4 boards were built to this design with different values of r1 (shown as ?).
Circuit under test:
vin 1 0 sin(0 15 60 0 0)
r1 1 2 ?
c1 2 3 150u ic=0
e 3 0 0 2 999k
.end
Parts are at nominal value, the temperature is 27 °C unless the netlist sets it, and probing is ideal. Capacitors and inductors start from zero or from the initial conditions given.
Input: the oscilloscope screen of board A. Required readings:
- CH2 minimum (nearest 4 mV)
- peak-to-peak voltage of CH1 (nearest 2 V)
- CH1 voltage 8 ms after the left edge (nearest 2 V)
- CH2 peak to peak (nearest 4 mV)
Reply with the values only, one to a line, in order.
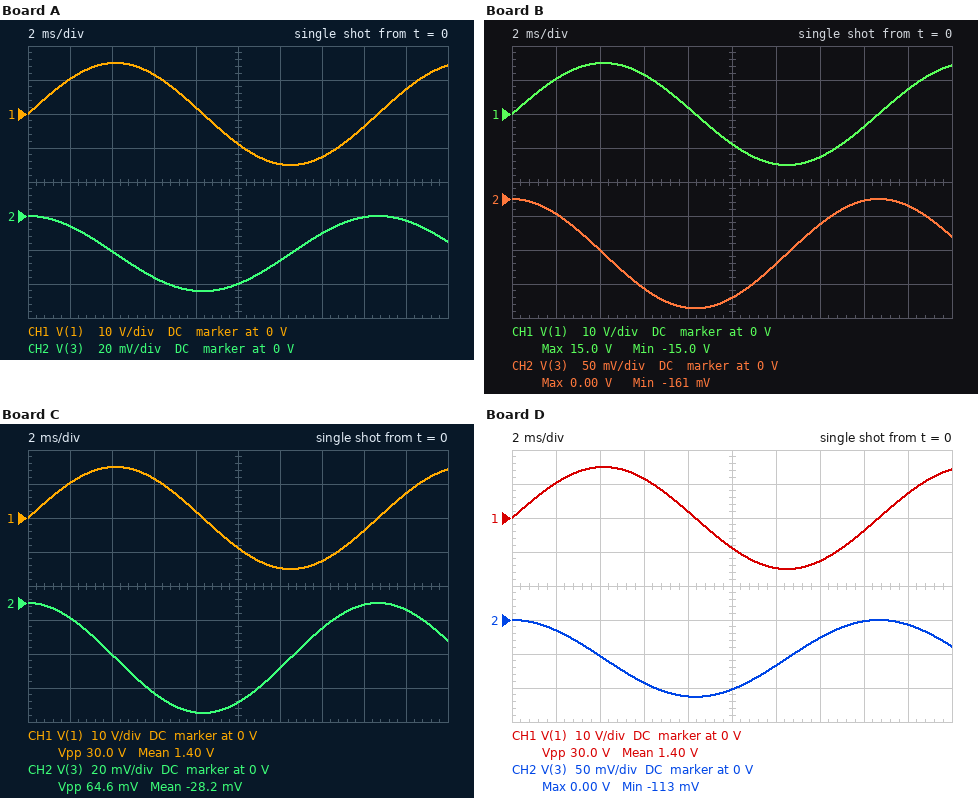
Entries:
-44 mV
30 V
2 V
44 mV
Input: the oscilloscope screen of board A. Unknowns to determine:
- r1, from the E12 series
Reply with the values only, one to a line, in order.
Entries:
12 kΩ
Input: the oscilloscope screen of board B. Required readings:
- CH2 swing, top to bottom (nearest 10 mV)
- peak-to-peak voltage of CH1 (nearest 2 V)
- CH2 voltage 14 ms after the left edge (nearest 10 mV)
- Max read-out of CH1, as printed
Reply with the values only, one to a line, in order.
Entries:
160 mV
30 V
-40 mV
15.0 V
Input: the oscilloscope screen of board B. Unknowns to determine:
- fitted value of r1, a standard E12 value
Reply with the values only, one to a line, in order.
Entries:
3.3 kΩ
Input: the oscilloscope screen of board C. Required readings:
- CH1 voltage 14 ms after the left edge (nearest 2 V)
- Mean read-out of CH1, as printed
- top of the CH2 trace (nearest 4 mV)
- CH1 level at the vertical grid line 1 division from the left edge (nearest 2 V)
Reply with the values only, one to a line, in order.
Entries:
-12 V
1.40 V
0 V
10 V
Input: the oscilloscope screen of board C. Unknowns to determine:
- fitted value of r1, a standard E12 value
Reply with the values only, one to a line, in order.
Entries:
8.2 kΩ
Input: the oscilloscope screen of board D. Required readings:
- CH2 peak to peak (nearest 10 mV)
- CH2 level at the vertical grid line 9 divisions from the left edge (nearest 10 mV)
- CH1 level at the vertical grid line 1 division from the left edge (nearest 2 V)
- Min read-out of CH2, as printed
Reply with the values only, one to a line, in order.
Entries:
110 mV
-10 mV
10 V
-113 mV
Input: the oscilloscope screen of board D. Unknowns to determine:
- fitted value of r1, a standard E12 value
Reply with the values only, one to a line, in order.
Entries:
4.7 kΩ
